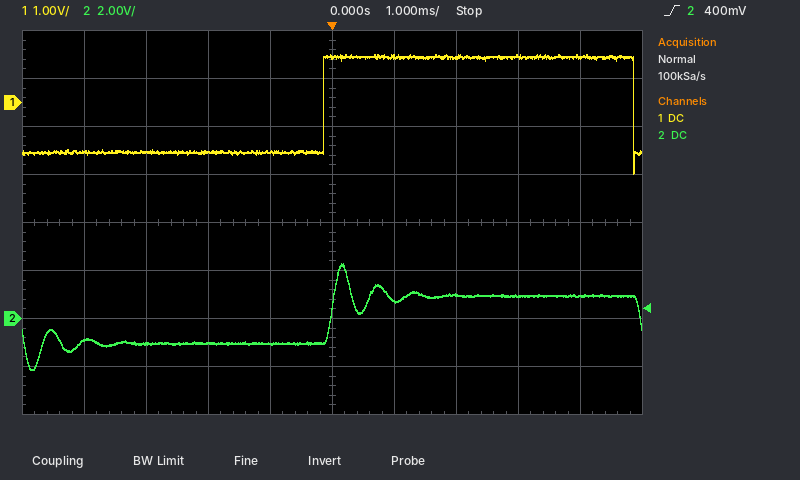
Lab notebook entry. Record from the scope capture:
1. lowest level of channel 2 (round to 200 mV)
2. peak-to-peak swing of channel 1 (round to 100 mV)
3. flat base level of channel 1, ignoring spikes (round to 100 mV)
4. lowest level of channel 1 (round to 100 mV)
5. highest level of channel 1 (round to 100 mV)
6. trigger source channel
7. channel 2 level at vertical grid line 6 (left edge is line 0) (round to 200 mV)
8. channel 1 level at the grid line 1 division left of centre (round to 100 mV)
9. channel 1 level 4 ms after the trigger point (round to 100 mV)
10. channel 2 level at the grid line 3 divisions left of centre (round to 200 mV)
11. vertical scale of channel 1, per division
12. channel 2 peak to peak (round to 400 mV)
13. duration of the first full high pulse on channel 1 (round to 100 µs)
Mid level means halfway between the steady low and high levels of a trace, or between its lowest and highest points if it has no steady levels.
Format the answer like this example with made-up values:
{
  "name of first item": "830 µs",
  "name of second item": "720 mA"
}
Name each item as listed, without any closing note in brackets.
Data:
{
  "lowest level of channel 2": "-2.2 V",
  "peak-to-peak swing of channel 1": "2.5 V",
  "flat base level of channel 1, ignoring spikes": "-1.0 V",
  "lowest level of channel 1": "-1.5 V",
  "highest level of channel 1": "1.0 V",
  "trigger source channel": "channel 2",
  "channel 2 level at vertical grid line 6 (left edge is line 0)": "800 mV",
  "channel 1 level at the grid line 1 division left of centre": "-1.0 V",
  "channel 1 level 4 ms after the trigger point": "1.0 V",
  "channel 2 level at the grid line 3 divisions left of centre": "-1.0 V",
  "vertical scale of channel 1, per division": "1 V",
  "channel 2 peak to peak": "4.4 V",
  "duration of the first full high pulse on channel 1": "5.0 ms"
}
